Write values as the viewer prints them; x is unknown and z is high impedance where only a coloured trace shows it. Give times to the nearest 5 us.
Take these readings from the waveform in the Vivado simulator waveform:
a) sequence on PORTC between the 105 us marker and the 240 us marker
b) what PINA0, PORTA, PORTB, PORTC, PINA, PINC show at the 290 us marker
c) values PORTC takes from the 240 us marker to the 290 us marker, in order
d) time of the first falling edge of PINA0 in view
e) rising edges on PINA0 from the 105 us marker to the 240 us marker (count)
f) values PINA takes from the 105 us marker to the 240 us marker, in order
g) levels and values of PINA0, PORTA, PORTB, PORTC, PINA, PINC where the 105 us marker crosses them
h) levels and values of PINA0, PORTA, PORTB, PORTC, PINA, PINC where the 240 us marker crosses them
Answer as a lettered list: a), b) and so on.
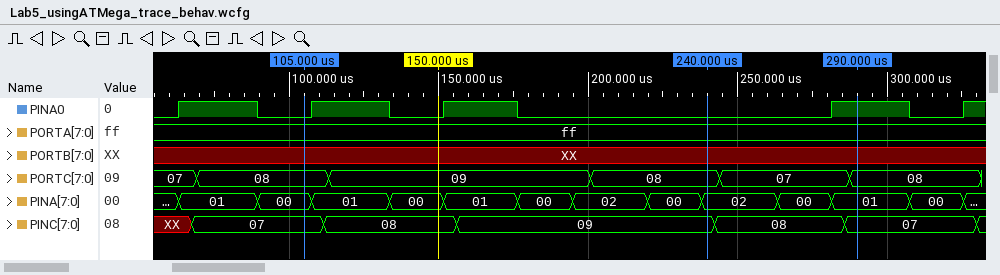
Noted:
a) 08, 09, 08
b) PINA0=1, PORTA=ff, PORTB=XX, PORTC=08, PINA=01, PINC=07
c) 08, 07, 08
d) 90 us
e) 2
f) 00, 01, 00, 01, 00, 02, 00, 02
g) PINA0=0, PORTA=ff, PORTB=XX, PORTC=08, PINA=00, PINC=07
h) PINA0=0, PORTA=ff, PORTB=XX, PORTC=08, PINA=02, PINC=09
